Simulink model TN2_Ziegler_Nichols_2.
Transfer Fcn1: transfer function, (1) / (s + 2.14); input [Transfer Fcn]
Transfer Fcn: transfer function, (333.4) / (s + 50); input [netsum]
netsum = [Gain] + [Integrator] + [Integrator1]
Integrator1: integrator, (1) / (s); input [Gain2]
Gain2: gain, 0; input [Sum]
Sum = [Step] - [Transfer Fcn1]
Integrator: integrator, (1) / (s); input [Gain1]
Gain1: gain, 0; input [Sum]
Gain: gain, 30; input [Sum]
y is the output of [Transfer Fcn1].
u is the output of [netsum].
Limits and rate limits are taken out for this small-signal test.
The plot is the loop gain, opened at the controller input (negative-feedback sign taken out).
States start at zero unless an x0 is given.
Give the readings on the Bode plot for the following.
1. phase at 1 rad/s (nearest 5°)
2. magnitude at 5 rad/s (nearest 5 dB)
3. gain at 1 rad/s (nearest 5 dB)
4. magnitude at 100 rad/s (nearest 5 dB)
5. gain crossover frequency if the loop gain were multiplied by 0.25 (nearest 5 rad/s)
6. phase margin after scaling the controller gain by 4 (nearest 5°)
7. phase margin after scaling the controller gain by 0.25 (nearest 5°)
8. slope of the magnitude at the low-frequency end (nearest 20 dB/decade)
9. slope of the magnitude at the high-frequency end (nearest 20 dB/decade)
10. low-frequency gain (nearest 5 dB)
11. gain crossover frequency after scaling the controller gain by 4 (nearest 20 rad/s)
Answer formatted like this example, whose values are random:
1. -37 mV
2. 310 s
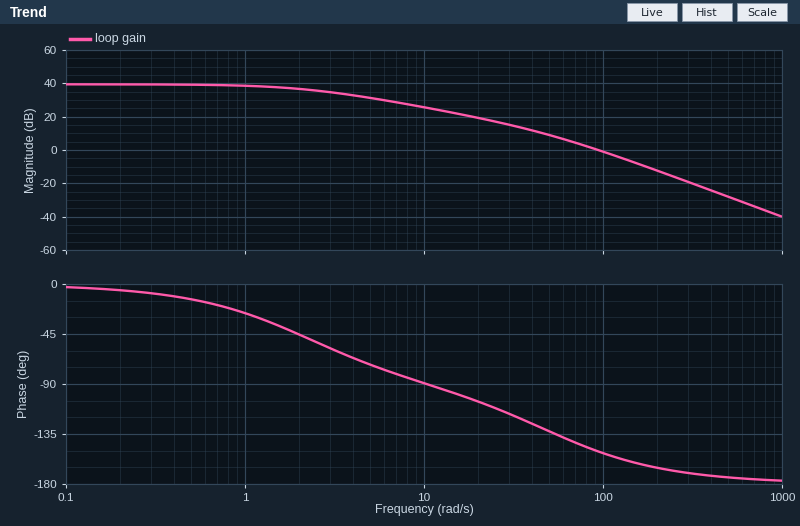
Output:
1. -25°
2. 30 dB
3. 40 dB
4. 0 dB
5. 40 rad/s
6. 15°
7. 55°
8. 0 dB/decade
9. -40 dB/decade
10. 40 dB
11. 200 rad/s
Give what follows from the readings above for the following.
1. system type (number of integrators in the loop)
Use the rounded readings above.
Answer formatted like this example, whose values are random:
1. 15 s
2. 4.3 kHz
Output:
1. 0
